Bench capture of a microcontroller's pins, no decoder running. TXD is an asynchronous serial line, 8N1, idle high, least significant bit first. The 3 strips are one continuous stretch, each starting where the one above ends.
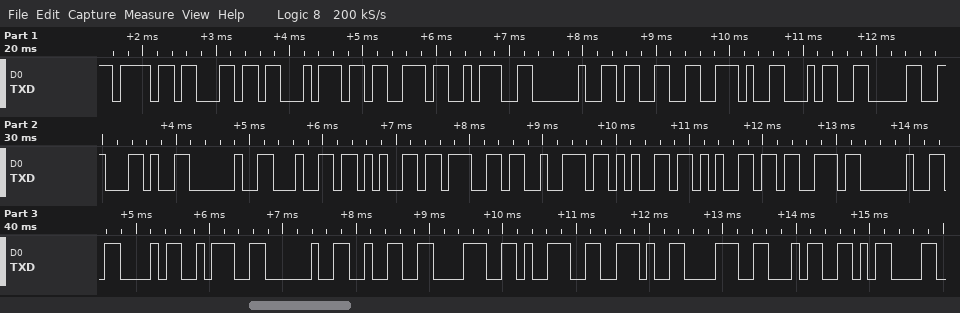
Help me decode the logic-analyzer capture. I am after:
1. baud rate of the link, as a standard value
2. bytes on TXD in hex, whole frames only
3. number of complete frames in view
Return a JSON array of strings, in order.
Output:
["9600 baud", "6F 6C 74 73 3A 20 33 2E 34 30 2C 20 64 65 67 72 65 65 73 20 43 3A 20 32 38 39 2E 38 34 0D", "30"]
